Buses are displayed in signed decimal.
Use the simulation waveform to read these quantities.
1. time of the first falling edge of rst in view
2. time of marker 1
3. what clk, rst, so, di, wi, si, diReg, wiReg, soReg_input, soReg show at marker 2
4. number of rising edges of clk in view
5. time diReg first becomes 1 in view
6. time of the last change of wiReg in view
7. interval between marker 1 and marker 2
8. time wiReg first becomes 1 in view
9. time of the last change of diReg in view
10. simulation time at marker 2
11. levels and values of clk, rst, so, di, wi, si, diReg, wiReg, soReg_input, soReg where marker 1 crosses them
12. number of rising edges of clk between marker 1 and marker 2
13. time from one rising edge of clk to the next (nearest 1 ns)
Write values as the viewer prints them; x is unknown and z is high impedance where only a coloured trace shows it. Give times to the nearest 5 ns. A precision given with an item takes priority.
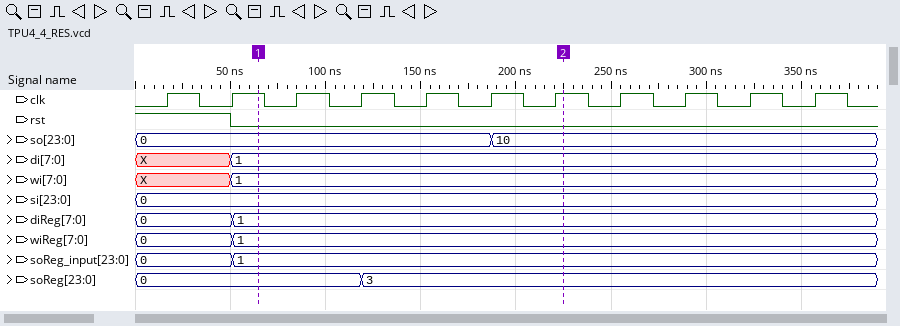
50 ns
65 ns
clk=1, rst=0, so=10, di=1, wi=1, si=0, diReg=1, wiReg=1, soReg_input=1, soReg=3
11
50 ns
50 ns
160 ns
50 ns
50 ns
225 ns
clk=1, rst=0, so=0, di=1, wi=1, si=0, diReg=1, wiReg=1, soReg_input=1, soReg=0
5
34 ns
